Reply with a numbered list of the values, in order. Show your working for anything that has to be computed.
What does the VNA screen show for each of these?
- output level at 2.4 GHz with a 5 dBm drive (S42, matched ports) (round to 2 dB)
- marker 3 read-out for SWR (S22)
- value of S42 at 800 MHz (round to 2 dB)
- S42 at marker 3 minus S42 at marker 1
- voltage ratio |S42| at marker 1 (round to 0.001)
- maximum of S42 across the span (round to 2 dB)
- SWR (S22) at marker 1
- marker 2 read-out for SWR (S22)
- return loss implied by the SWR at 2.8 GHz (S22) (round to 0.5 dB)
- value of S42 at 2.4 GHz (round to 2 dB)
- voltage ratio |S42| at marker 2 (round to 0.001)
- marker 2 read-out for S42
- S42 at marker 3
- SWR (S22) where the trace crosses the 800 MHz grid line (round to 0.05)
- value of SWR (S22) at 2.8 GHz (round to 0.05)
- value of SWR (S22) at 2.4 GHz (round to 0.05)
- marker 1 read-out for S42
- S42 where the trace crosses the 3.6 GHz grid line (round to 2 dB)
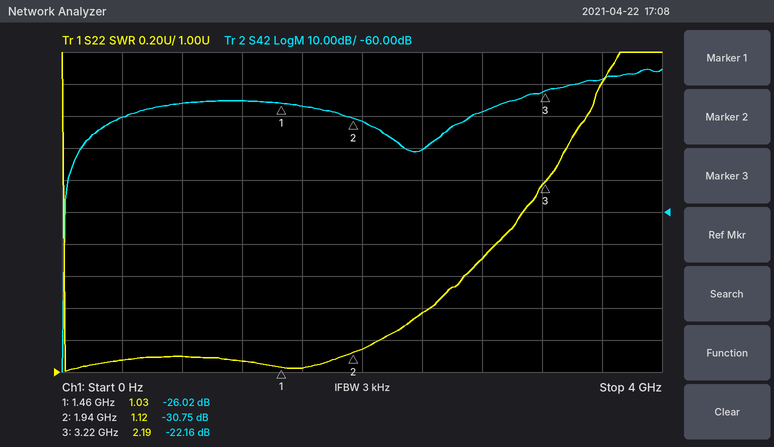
1. 5 dBm + (-40 dB) = -36 dBm
2. 2.19
3. -26 dB
4. -22.16 − (-26.02) = 3.86 dB
5. 10^(-26.02/20) ≈ 0.050
6. -16 dB
7. 1.03
8. 1.12
9. −20 log10((1.7 − 1)/(1.7 + 1)) ≈ 11.7 dB, so 11.5 dB to the nearest 0.5 dB
10. -40 dB
11. 10^(-30.75/20) ≈ 0.029
12. -30.75 dB
13. -22.16 dB
14. 1.10
15. 1.70
16. 1.35
17. -26.02 dB
18. -18 dB
